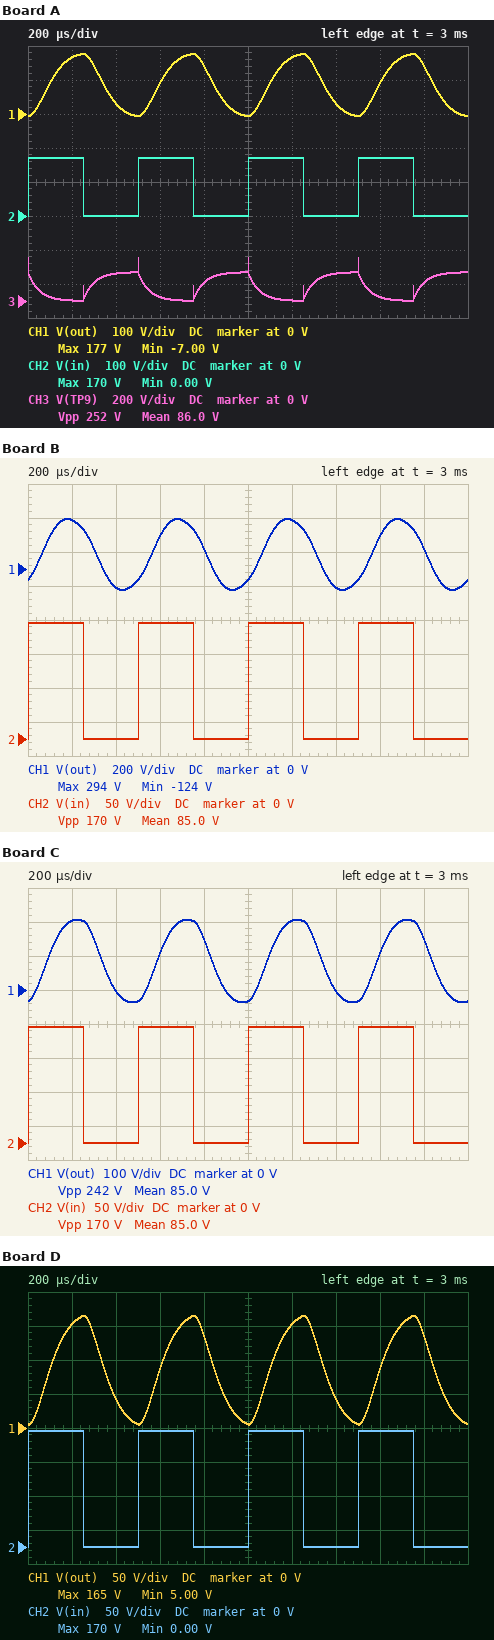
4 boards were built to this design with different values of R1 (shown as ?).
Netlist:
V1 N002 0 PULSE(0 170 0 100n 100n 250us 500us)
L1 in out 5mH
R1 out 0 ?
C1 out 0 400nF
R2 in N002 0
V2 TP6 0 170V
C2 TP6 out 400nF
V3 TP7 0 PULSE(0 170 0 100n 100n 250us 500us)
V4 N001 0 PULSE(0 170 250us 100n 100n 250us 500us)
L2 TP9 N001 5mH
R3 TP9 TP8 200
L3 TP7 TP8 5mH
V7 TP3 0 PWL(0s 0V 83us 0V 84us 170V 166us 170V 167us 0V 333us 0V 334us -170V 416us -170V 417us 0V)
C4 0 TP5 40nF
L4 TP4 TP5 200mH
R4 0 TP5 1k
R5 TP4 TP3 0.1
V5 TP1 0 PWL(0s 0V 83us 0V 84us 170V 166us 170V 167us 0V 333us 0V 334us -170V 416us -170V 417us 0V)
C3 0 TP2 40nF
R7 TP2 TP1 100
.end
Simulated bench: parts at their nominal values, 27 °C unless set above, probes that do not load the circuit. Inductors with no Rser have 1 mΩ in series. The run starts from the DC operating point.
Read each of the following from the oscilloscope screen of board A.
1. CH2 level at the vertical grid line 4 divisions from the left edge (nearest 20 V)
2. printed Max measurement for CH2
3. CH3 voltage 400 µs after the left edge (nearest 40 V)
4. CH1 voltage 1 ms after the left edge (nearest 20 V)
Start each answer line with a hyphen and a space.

- 0 V
- 170 V
- 160 V
- 0 V
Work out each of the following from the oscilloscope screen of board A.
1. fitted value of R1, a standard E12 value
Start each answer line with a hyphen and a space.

- 56 Ω
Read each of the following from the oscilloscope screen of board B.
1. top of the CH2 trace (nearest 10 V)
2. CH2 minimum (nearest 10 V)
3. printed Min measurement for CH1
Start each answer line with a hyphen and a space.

- 170 V
- 0 V
- -124 V
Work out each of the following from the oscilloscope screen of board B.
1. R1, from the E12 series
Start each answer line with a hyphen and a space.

- 180 Ω
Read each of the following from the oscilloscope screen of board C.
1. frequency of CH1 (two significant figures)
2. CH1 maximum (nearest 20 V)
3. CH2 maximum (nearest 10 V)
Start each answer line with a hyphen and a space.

- 2.0 kHz
- 200 V
- 170 V
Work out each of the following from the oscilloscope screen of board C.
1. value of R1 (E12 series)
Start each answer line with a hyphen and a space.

- 82 Ω
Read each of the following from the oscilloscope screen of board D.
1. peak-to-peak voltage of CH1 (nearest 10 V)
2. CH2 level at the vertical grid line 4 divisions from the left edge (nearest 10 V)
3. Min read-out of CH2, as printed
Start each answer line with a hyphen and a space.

- 160 V
- 0 V
- 0.00 V
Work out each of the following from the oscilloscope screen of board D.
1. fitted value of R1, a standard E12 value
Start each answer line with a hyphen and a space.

- 47 Ω
